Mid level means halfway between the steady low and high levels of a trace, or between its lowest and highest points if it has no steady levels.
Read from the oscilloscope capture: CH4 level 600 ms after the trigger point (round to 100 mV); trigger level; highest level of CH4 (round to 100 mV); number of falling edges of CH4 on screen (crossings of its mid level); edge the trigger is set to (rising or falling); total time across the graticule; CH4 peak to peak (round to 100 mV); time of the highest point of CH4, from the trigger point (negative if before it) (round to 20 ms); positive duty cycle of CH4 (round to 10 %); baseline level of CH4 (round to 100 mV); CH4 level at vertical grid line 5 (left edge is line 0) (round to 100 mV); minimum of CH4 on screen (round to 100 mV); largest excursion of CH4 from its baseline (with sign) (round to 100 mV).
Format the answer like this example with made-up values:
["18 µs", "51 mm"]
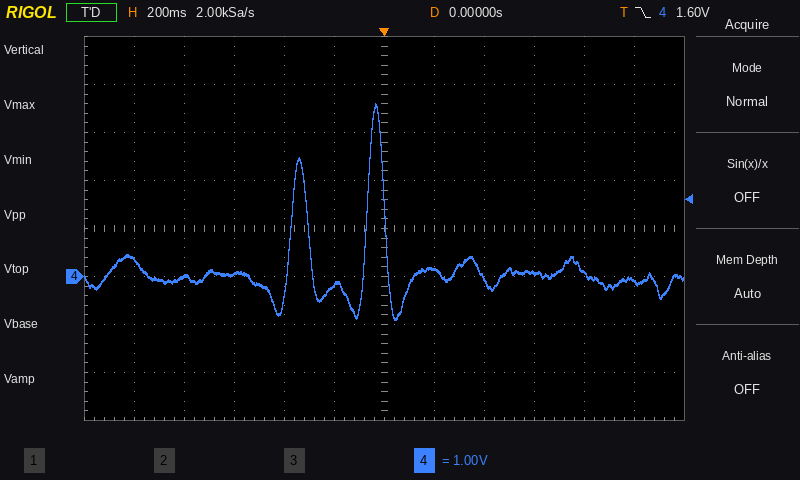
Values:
["100 mV", "1.60 V", "3.6 V", "2", "falling", "2.4 s", "4.5 V", "-40 ms", "20 %", "0.0 V", "-200 mV", "-900 mV", "+3.6 V"]
